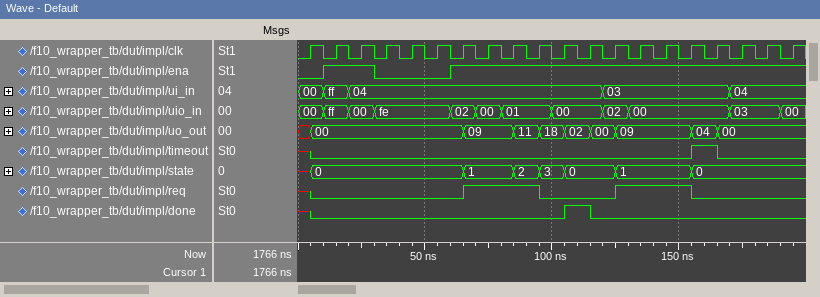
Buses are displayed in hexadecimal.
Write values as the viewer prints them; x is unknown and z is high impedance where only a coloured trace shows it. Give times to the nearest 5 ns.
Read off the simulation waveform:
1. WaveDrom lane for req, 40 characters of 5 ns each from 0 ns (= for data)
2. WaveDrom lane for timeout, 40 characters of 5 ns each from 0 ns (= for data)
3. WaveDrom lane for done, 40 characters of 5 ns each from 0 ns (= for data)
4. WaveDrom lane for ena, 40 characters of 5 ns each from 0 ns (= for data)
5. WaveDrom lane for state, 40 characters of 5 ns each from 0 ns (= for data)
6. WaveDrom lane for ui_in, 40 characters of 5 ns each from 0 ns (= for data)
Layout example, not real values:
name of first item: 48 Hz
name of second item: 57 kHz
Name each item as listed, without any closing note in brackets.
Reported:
WaveDrom lane for req, 40 characters of 5 ns each from 0 ns: {name: 'req', wave: 'x0...........1.....0.....1.....0........'}
WaveDrom lane for timeout, 40 characters of 5 ns each from 0 ns: {name: 'timeout', wave: 'x0.............................1.0......'}
WaveDrom lane for done, 40 characters of 5 ns each from 0 ns: {name: 'done', wave: 'x0...................1.0................'}
WaveDrom lane for ena, 40 characters of 5 ns each from 0 ns: {name: 'ena', wave: '0.1...0.....1...........................'}
WaveDrom lane for state, 40 characters of 5 ns each from 0 ns: {name: 'state', wave: 'x=...........=...=.=.=...=.....=........', data: '0 1 2 3 0 1 0'}
WaveDrom lane for ui_in, 40 characters of 5 ns each from 0 ns: {name: 'ui_in', wave: '=.=.=...................=.........=.....', data: '00 ff 04 03 04'}
